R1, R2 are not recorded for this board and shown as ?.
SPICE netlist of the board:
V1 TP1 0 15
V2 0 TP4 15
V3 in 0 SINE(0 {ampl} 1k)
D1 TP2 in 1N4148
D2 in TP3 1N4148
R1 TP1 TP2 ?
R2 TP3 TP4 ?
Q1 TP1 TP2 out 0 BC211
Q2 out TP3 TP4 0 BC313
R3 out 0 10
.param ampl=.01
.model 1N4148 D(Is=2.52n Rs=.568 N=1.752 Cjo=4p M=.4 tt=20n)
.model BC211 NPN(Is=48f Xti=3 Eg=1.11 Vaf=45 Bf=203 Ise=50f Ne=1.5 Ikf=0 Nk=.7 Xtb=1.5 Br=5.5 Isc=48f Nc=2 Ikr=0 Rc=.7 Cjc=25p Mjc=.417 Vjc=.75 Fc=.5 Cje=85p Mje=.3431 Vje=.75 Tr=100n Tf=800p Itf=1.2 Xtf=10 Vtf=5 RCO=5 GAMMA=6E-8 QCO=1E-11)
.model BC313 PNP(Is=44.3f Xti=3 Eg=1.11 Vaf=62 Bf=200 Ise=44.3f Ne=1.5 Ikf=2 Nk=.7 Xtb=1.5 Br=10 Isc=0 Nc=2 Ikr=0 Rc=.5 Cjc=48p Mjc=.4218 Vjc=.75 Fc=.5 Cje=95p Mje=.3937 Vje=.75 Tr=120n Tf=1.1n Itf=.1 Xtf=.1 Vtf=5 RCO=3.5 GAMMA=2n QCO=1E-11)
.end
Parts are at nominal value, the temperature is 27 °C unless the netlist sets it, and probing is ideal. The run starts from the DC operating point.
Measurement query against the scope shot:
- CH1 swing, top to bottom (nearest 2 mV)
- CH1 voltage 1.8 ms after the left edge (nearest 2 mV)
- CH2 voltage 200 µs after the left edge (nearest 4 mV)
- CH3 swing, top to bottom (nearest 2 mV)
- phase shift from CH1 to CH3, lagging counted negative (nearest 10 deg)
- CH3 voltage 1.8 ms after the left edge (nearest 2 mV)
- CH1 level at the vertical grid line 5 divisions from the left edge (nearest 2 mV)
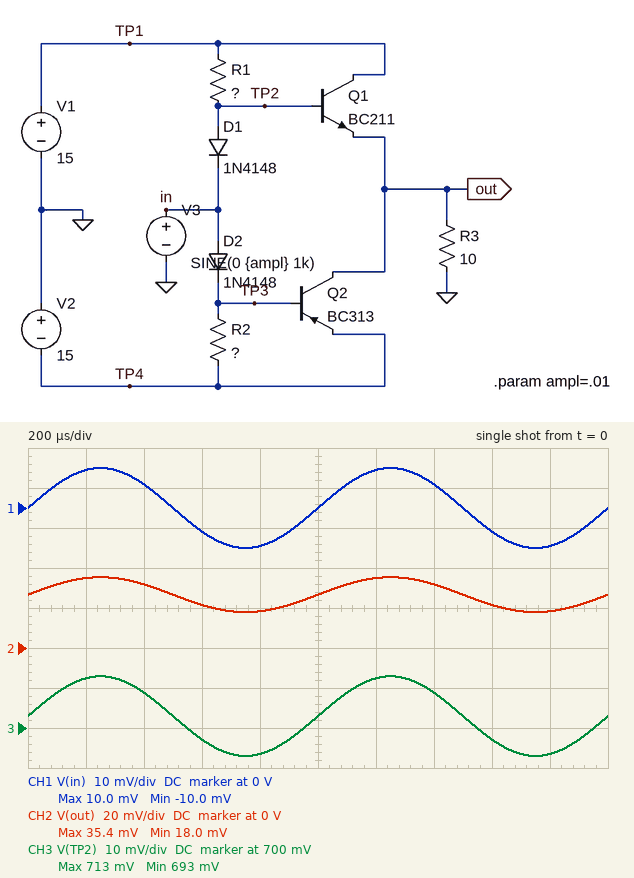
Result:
20 mV
-10 mV
36 mV
20 mV
0 deg
694 mV
0 V
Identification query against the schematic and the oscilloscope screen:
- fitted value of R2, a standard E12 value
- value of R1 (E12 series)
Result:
1.2 kΩ
1.2 kΩ
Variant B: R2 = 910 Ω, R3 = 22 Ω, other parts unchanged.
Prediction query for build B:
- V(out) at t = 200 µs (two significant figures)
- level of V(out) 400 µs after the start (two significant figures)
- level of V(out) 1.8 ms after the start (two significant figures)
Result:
34 mV
31 mV
16 mV
